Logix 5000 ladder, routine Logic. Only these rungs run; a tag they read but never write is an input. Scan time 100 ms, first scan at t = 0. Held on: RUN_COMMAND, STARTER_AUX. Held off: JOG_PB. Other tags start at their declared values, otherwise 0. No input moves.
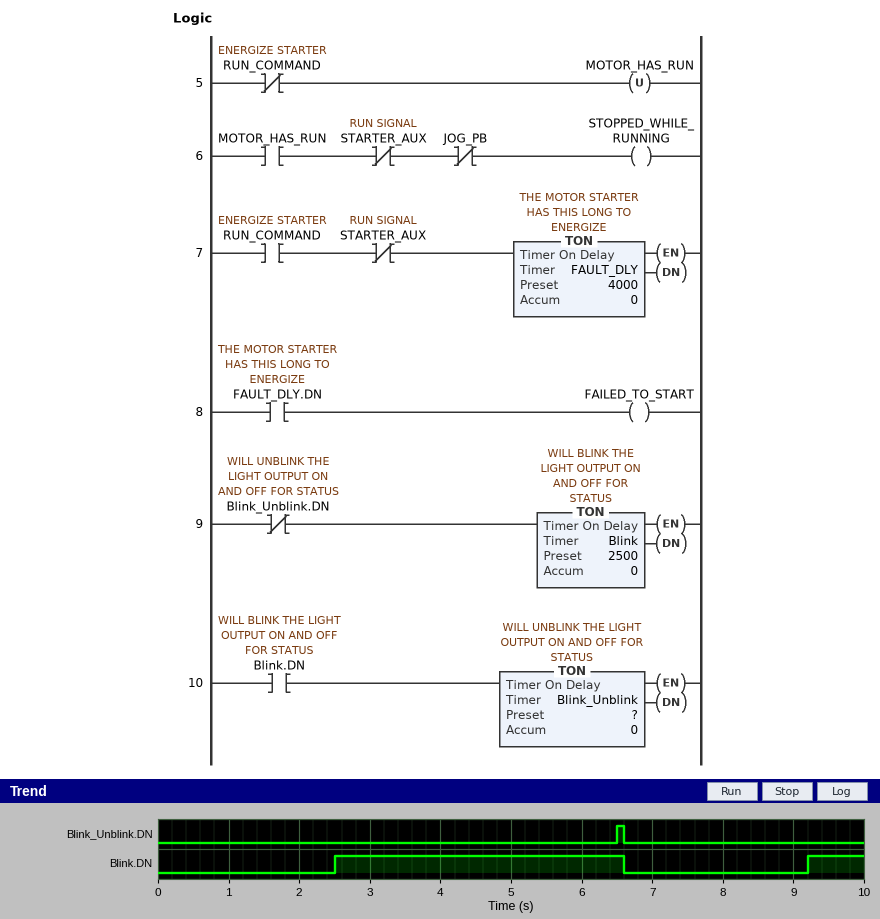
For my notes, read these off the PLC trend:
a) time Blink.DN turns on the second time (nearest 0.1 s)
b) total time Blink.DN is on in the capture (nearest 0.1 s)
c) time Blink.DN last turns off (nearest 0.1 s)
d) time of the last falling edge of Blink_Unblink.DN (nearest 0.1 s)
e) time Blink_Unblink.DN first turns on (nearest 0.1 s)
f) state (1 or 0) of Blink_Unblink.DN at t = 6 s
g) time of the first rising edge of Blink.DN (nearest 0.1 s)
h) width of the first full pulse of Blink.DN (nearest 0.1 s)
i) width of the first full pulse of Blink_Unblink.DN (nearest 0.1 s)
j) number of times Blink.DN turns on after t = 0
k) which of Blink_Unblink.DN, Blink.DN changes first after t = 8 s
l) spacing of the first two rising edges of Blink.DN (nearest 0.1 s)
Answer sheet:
9.2 s
4.9 s
6.6 s
6.6 s
6.5 s
0
2.5 s
4.1 s
0.1 s
2
Blink.DN
6.7 s
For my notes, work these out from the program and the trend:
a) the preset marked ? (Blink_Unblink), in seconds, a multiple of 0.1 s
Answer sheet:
4.0 s
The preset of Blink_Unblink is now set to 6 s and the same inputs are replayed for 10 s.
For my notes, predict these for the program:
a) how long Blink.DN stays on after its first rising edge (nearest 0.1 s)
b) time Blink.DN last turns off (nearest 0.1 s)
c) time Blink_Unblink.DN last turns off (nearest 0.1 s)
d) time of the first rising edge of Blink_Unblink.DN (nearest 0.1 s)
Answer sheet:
6.1 s
8.6 s
8.6 s
8.5 s
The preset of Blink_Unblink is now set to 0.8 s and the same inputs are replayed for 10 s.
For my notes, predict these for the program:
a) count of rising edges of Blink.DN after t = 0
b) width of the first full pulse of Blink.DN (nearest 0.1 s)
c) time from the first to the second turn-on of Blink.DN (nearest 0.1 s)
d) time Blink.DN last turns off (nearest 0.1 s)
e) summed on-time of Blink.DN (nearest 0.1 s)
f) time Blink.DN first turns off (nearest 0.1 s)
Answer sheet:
3
0.9 s
3.5 s
6.9 s
2.3 s
3.4 s
